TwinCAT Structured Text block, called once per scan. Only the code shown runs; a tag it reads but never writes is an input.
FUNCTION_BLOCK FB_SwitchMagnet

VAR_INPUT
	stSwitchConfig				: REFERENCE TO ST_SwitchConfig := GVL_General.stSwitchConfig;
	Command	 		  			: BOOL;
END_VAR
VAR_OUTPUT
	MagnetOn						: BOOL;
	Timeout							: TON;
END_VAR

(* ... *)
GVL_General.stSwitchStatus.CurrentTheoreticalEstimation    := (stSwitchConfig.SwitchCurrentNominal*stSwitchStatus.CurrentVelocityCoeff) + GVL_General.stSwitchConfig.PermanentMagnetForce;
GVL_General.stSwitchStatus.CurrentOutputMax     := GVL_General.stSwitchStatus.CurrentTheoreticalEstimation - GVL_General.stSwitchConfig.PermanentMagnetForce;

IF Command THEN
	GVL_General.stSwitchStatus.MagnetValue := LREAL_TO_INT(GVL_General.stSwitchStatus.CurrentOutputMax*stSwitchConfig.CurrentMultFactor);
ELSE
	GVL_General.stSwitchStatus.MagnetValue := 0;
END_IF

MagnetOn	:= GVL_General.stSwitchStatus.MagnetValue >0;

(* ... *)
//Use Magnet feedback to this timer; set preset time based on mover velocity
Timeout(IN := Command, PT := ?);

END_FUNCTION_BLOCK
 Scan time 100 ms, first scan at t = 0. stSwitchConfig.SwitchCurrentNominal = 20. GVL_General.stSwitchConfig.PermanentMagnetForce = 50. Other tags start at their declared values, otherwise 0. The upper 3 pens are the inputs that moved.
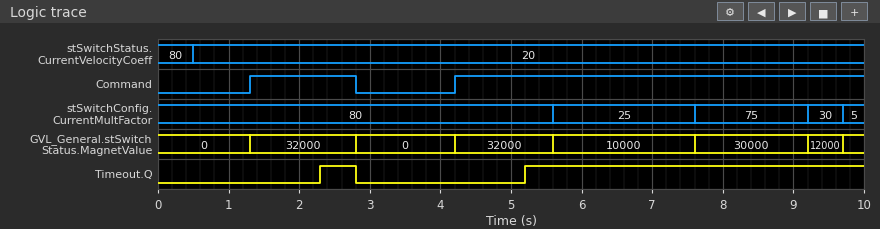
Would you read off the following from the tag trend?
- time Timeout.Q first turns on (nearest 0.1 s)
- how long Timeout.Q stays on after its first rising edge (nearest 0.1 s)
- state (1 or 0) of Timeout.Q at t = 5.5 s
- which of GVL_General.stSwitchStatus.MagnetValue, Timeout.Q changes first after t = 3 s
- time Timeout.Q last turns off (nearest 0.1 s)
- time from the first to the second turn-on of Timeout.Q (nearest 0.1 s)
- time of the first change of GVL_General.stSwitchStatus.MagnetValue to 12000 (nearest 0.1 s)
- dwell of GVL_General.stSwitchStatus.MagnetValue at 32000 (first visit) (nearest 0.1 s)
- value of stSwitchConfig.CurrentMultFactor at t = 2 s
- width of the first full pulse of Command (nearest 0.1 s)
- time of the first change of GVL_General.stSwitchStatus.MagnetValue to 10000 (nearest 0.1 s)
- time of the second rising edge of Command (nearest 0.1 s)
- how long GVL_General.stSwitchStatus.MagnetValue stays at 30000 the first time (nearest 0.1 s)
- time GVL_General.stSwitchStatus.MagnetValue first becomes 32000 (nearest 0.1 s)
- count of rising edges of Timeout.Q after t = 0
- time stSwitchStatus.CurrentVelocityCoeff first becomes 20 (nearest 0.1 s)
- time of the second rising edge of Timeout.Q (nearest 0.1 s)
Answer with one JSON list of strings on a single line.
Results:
["2.3 s", "0.5 s", "1", "GVL_General.stSwitchStatus.MagnetValue", "2.8 s", "2.9 s", "9.2 s", "1.5 s", "80", "1.5 s", "5.6 s", "4.2 s", "1.6 s", "1.3 s", "2", "0.5 s", "5.2 s"]
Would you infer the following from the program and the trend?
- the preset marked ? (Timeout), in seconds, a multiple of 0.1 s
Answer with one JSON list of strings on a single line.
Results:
["1.0 s"]
